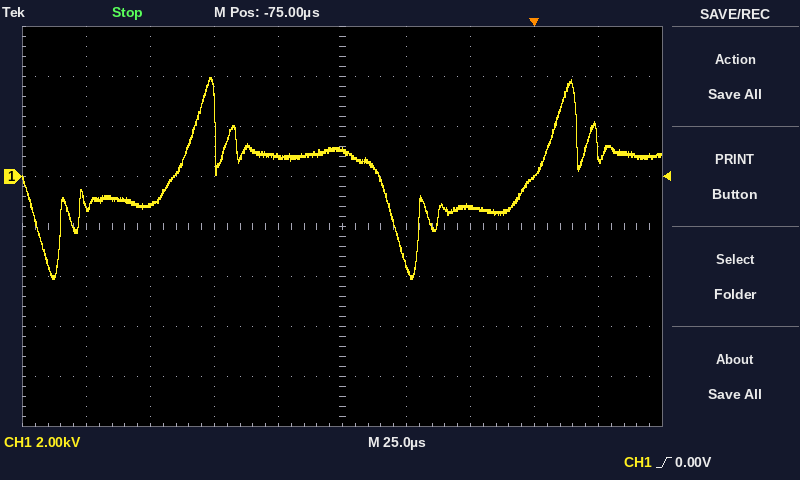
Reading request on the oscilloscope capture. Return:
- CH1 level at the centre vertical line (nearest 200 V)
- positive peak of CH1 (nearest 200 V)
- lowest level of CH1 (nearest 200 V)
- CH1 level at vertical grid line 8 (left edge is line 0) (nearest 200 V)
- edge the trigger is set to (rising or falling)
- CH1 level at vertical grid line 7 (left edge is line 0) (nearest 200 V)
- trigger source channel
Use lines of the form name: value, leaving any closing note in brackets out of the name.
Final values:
CH1 level at the centre vertical line: 1.0 kV
positive peak of CH1: 4.0 kV
lowest level of CH1: -4.2 kV
CH1 level at vertical grid line 8 (left edge is line 0): 0.0 kV
edge the trigger is set to: rising
CH1 level at vertical grid line 7 (left edge is line 0): -1.2 kV
trigger source channel: CH1
